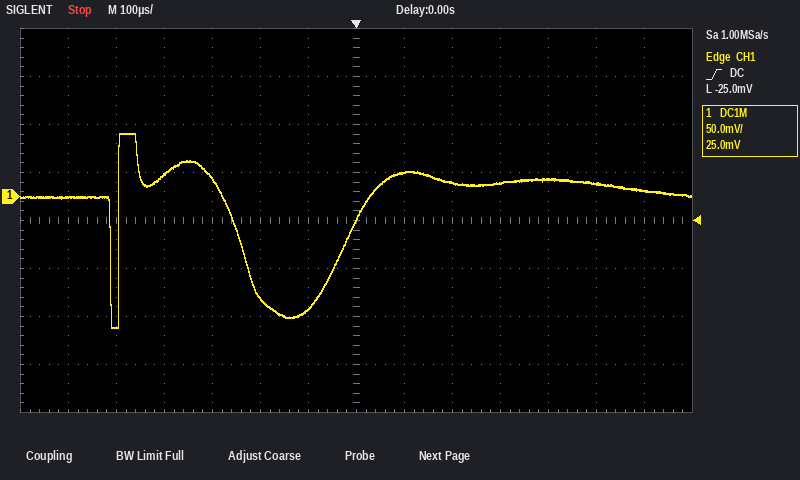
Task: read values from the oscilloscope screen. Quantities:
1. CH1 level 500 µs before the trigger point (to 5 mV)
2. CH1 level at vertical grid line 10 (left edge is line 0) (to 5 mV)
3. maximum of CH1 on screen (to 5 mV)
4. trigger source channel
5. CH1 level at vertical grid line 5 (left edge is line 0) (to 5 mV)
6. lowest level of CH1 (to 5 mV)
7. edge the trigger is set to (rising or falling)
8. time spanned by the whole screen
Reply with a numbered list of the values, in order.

1. -135 mV
2. 15 mV
3. 65 mV
4. CH1
5. -105 mV
6. -135 mV
7. rising
8. 1.4 ms
